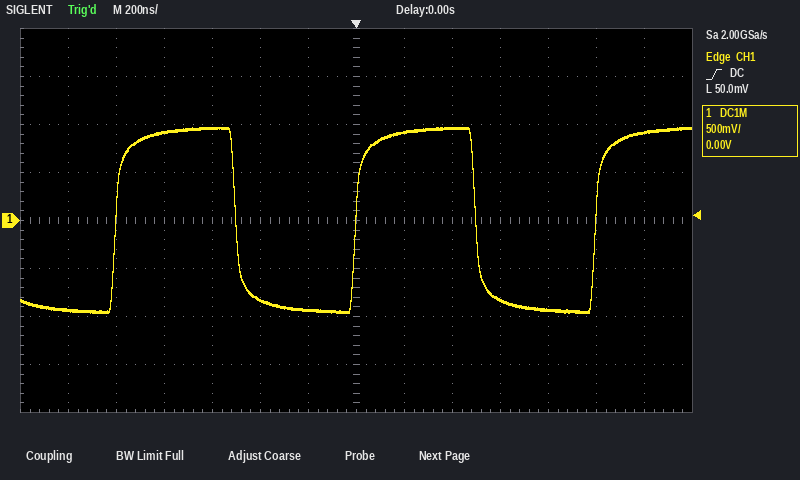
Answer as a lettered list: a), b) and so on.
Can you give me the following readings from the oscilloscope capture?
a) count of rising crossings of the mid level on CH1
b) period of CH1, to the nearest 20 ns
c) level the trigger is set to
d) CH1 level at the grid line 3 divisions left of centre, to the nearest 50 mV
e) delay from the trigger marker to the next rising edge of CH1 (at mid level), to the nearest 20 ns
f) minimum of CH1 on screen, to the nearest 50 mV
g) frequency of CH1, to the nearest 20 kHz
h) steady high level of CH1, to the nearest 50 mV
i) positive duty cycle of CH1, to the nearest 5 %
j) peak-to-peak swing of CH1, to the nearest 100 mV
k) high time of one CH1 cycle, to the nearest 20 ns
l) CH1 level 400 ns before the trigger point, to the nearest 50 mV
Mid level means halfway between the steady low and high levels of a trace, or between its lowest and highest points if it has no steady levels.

a) 3
b) 1.00 µs
c) 50.0 mV
d) 950 mV
e) 1.00 µs
f) -950 mV
g) 1.00 MHz
h) 950 mV
i) 50 %
j) 1.90 V
k) 500 ns
l) -850 mV
